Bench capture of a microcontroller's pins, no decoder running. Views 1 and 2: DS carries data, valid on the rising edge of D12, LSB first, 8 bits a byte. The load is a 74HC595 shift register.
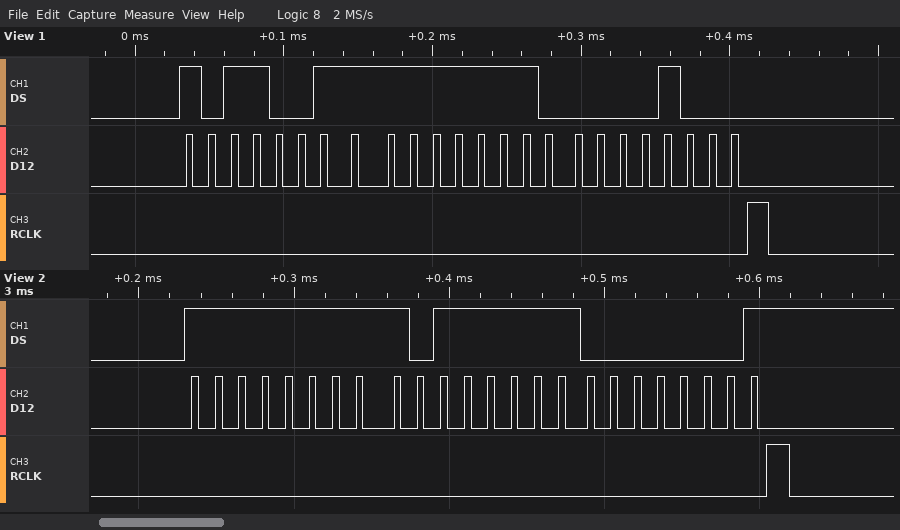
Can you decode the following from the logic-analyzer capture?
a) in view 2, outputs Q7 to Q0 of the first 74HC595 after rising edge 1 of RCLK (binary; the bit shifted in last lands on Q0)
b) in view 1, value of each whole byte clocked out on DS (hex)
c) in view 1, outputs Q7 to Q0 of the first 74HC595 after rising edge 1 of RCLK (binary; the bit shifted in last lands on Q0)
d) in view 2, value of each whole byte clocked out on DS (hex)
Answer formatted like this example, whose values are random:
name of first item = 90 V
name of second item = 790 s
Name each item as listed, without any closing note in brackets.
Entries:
in view 2, outputs Q7 to Q0 of the first 74HC595 after rising edge 1 of RCLK = 00000001
in view 1, value of each whole byte clocked out on DS = CD 7F 10
in view 1, outputs Q7 to Q0 of the first 74HC595 after rising edge 1 of RCLK = 00001000
in view 2, value of each whole byte clocked out on DS = 0xFF 0xFD 0x80
